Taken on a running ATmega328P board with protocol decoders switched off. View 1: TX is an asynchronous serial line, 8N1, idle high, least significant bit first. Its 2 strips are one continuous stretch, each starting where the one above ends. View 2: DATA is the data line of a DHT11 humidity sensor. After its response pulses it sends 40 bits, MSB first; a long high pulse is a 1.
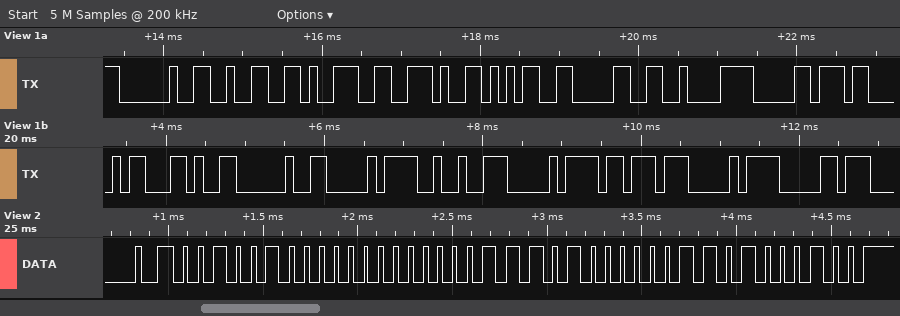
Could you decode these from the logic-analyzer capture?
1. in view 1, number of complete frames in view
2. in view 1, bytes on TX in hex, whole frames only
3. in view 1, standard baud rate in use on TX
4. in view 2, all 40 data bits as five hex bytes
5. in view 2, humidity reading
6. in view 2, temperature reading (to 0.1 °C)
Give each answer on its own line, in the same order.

17
20 32 39 2E 35 30 C2 B0 43 2C 20 D0 92 D0 BB D0 B0
9600 baud
24 00 1D 03 44
36 %
29.3 °C
